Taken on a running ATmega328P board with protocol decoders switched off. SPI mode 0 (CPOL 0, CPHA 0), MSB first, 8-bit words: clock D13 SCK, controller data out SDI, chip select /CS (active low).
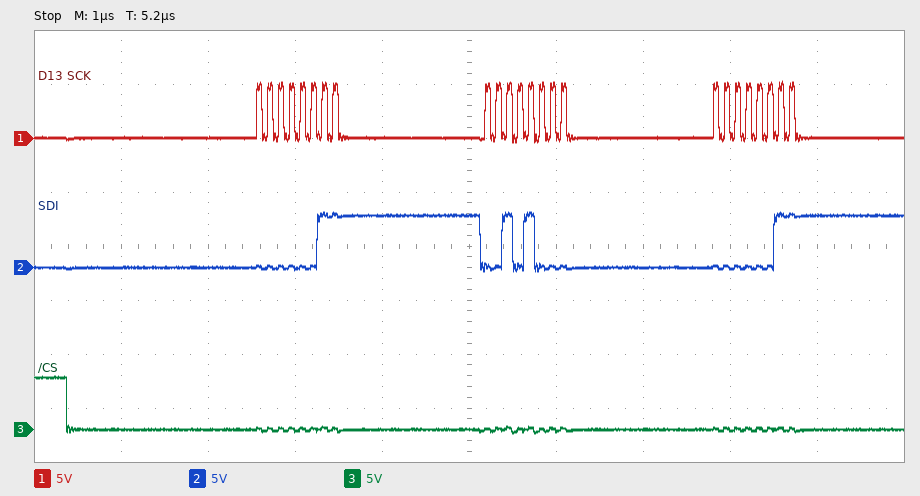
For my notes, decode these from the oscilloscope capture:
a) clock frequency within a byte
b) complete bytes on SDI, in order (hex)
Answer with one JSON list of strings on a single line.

["8 MHz", "03 28 03"]
